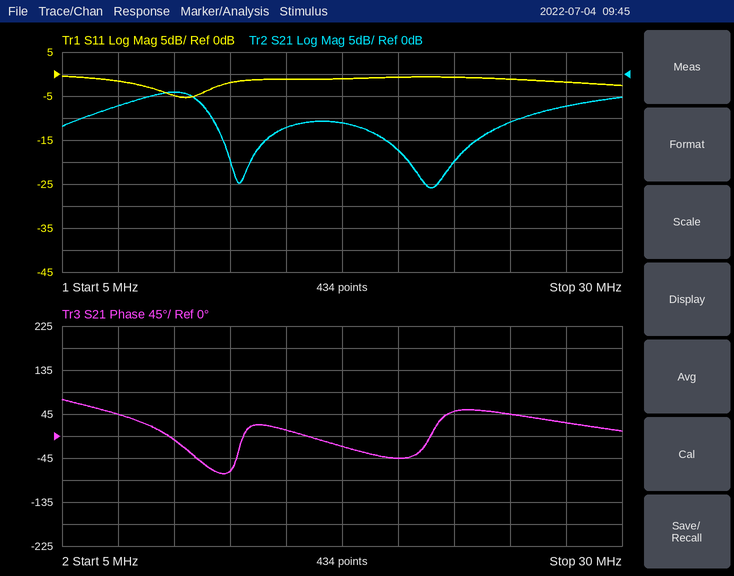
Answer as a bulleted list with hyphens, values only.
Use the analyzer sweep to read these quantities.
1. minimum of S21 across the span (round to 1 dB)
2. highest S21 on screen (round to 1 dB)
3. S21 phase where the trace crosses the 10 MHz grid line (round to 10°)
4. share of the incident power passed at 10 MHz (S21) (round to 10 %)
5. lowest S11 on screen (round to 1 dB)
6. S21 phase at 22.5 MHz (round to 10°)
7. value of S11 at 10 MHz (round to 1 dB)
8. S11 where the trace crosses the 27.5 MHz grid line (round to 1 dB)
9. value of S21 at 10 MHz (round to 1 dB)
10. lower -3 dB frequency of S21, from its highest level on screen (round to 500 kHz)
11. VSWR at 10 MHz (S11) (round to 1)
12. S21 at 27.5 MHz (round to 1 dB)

- -26 dB
- -4 dB
- -10°
- 40 %
- -5 dB
- 50°
- -5 dB
- -2 dB
- -4 dB
- 7.5 MHz
- 4
- -7 dB
